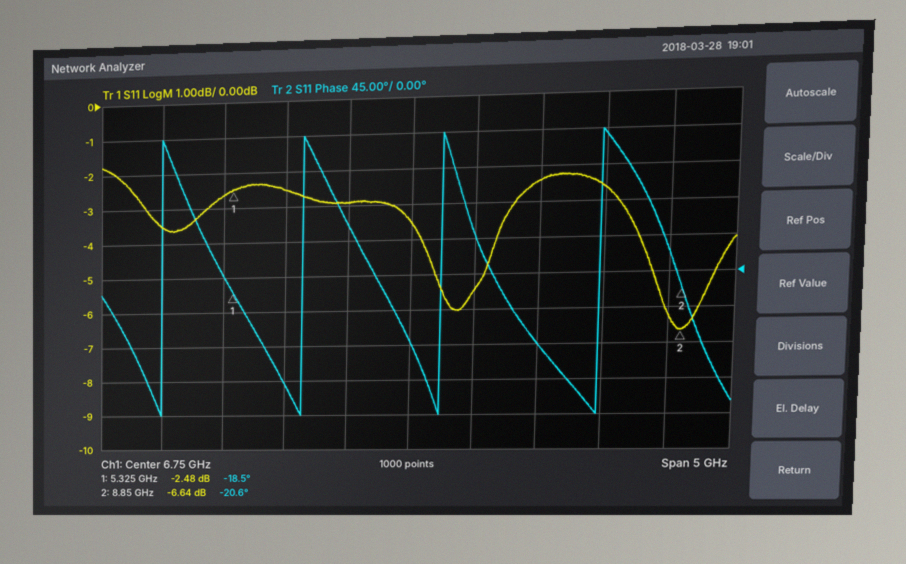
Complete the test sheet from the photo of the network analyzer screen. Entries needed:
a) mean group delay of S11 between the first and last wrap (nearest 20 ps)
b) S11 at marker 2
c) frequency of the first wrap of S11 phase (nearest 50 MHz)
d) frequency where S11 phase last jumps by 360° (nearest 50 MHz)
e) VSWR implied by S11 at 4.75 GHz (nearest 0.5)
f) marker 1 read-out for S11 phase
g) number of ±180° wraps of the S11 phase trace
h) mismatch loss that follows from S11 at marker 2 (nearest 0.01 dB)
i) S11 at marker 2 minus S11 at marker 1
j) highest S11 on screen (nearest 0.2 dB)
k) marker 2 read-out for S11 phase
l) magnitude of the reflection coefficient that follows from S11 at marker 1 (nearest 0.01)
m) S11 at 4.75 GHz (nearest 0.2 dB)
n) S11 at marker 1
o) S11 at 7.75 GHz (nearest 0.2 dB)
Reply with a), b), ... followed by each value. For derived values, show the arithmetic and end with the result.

a) 3 cycles / (8.20 GHz − 4.75 GHz) ≈ 870 ps, so 860 ps to the nearest 20 ps
b) -6.64 dB
c) 4.75 GHz
d) 8.20 GHz
e) |Γ| = 10^(-3.6/20) = 0.6607; VSWR = (1 + 0.6607)/(1 − 0.6607) ≈ 4.89, so 5.0 to the nearest 0.5
f) -18.5°
g) 4
h) −10 log10(1 − 10^(-6.64/10)) ≈ 1.06 dB
i) -6.64 − (-2.48) = -4.16 dB
j) -1.8 dB
k) -20.6°
l) 10^(-2.48/20) ≈ 0.75
m) -3.6 dB
n) -2.48 dB
o) -2.4 dB
